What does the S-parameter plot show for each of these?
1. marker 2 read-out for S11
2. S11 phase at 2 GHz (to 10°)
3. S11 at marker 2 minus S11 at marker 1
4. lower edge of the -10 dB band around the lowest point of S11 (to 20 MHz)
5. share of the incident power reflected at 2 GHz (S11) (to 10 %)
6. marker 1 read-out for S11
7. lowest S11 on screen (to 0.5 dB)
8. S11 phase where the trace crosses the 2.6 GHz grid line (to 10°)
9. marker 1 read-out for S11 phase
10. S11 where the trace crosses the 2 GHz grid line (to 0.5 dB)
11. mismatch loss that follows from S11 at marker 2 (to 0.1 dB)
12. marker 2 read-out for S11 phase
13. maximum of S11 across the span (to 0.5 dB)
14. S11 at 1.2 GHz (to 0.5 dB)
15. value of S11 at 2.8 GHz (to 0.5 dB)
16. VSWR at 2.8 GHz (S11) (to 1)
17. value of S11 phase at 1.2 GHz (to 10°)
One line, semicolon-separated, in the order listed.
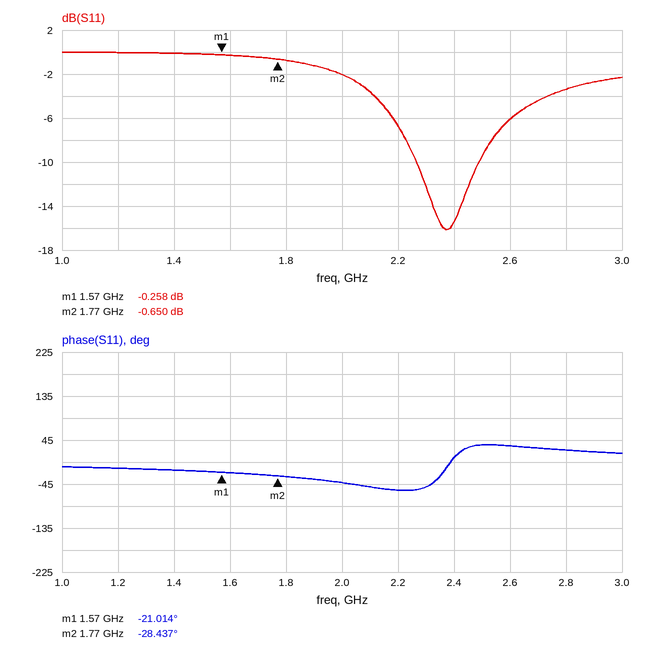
-0.650 dB; -40°; -0.392 dB; 2.26 GHz; 60 %; -0.258 dB; -16.0 dB; 30°; -21.014°; -2.0 dB; 8.6 dB; -28.437°; 0.0 dB; 0.0 dB; -3.5 dB; 5; -10°
